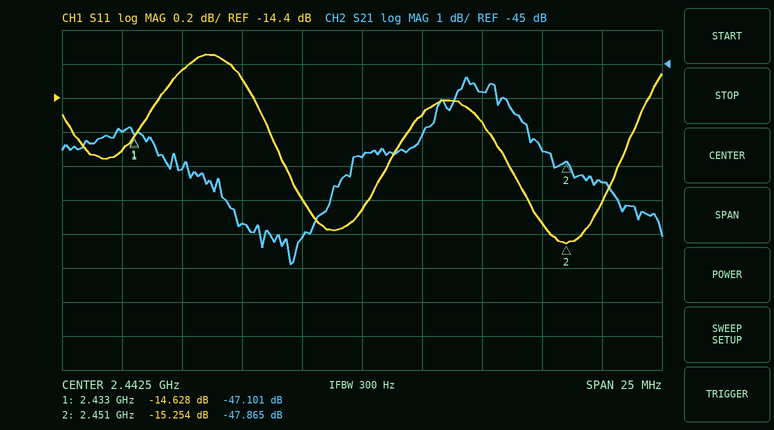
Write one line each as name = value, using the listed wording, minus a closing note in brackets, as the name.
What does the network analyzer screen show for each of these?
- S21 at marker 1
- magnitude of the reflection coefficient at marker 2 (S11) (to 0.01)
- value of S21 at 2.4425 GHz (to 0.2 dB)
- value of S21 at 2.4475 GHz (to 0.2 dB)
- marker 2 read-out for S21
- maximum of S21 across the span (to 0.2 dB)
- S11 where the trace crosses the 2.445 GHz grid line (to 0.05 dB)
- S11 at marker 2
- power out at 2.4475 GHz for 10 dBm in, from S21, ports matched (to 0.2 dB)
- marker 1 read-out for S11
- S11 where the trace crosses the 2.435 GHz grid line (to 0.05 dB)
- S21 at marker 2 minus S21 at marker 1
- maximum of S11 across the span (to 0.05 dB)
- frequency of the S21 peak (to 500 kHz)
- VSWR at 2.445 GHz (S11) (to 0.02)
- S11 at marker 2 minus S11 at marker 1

S21 at marker 1 = -47.101 dB
magnitude of the reflection coefficient at marker 2 (S11) = 0.17
value of S21 at 2.4425 GHz = -47.8 dB
value of S21 at 2.4475 GHz = -45.8 dB
marker 2 read-out for S21 = -47.865 dB
maximum of S21 across the span = -45.4 dB
S11 where the trace crosses the 2.445 GHz grid line = -14.50 dB
S11 at marker 2 = -15.254 dB
power out at 2.4475 GHz for 10 dBm in, from S21, ports matched = -35.8 dBm
marker 1 read-out for S11 = -14.628 dB
S11 where the trace crosses the 2.435 GHz grid line = -14.25 dB
S21 at marker 2 minus S21 at marker 1 = -0.764 dB
maximum of S11 across the span = -14.15 dB
frequency of the S21 peak = 2.4470 GHz
VSWR at 2.445 GHz (S11) = 1.46
S11 at marker 2 minus S11 at marker 1 = -0.626 dB
